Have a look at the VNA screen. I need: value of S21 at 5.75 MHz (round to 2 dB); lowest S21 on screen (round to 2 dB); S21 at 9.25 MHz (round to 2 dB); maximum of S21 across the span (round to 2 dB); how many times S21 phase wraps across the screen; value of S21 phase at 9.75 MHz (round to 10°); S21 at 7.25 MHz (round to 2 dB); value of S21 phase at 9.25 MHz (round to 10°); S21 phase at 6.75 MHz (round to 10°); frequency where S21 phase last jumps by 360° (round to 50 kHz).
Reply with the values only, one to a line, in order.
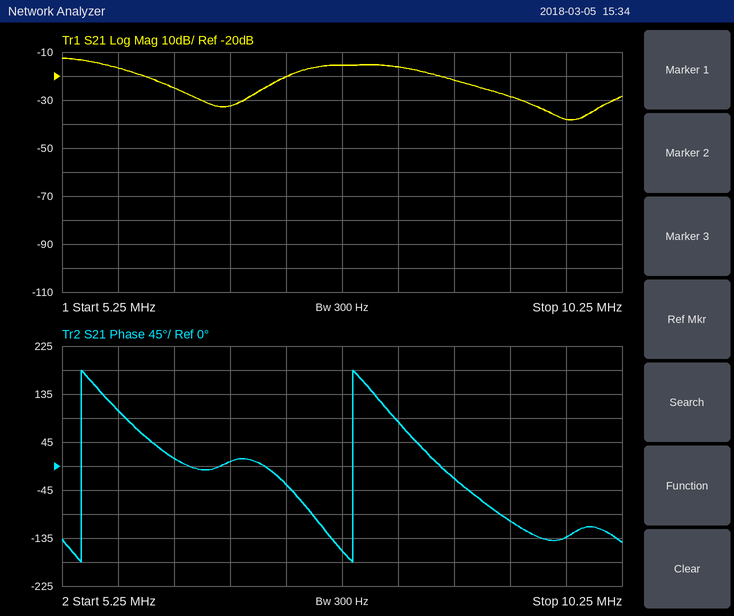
-16 dB
-38 dB
-28 dB
-12 dB
2
-130°
-20 dB
-100°
10°
7.85 MHz
